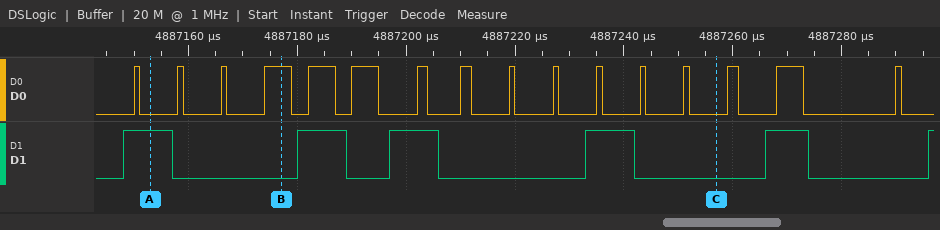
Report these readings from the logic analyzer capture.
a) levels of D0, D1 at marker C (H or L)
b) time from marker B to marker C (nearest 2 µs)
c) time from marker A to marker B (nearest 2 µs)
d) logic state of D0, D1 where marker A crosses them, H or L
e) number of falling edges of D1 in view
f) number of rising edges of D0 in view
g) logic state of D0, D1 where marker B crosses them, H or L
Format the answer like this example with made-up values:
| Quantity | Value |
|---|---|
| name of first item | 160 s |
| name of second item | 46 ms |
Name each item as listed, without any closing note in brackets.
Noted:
| Quantity | Value |
|---|---|
| levels of D0, D1 at marker C | D0=L, D1=L |
| time from marker B to marker C | 80 µs |
| time from marker A to marker B | 24 µs |
| logic state of D0, D1 where marker A crosses them, H or L | D0=L, D1=H |
| number of falling edges of D1 in view | 5 |
| number of rising edges of D0 in view | 16 |
| logic state of D0, D1 where marker B crosses them, H or L | D0=H, D1=L |
